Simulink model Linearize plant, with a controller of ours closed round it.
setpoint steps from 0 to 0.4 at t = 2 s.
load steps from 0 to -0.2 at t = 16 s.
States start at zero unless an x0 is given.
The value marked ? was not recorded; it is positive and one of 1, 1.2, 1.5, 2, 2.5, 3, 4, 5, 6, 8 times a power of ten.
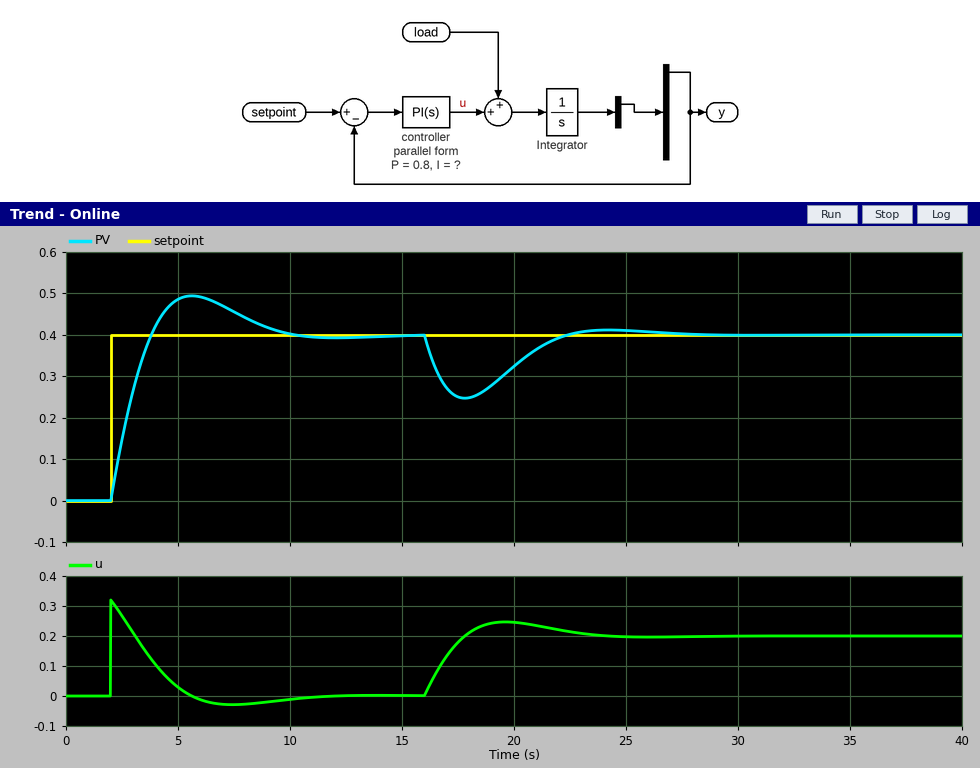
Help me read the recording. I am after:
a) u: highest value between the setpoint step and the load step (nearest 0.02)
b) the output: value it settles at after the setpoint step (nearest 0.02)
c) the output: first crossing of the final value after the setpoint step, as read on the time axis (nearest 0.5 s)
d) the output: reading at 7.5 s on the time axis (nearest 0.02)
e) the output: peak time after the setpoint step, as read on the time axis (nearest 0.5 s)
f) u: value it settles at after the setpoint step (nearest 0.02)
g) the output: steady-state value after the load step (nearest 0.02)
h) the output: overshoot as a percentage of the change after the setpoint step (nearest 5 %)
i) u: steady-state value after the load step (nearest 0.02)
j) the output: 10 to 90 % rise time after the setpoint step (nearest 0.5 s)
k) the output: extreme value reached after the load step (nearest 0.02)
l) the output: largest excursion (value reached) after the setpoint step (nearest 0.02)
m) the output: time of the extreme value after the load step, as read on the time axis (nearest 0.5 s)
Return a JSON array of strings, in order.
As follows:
["0.32", "0.40", "4.0 s", "0.46", "5.5 s", "0.00", "0.40", "25 %", "0.20", "1.5 s", "0.24", "0.50", "18.0 s"]
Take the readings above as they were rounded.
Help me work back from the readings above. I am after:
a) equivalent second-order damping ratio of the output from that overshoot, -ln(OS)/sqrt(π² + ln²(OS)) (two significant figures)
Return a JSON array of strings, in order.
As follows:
["0.40"]
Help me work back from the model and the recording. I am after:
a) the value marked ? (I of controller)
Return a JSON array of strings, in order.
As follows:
["0.4"]
